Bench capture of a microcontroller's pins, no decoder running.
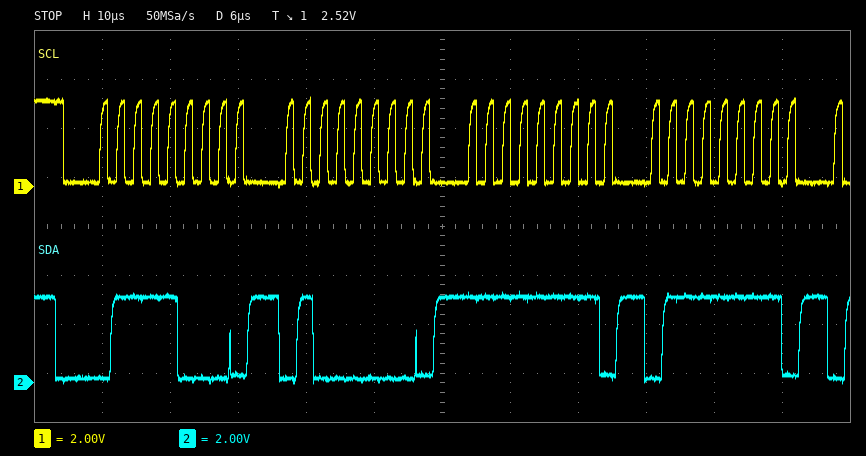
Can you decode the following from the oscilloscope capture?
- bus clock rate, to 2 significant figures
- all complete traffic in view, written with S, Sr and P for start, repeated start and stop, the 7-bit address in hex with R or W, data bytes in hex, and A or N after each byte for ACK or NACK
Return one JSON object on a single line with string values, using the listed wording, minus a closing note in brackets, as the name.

{"bus clock rate, to 2 significant figures": "400 kHz", "all complete traffic in view, written with S, Sr and P for start, repeated start and stop, the 7-bit address in hex with R or W, data bytes in hex, and A or N after each byte for ACK or NACK": "S 3CW A 40 A FF A 7F A"}
